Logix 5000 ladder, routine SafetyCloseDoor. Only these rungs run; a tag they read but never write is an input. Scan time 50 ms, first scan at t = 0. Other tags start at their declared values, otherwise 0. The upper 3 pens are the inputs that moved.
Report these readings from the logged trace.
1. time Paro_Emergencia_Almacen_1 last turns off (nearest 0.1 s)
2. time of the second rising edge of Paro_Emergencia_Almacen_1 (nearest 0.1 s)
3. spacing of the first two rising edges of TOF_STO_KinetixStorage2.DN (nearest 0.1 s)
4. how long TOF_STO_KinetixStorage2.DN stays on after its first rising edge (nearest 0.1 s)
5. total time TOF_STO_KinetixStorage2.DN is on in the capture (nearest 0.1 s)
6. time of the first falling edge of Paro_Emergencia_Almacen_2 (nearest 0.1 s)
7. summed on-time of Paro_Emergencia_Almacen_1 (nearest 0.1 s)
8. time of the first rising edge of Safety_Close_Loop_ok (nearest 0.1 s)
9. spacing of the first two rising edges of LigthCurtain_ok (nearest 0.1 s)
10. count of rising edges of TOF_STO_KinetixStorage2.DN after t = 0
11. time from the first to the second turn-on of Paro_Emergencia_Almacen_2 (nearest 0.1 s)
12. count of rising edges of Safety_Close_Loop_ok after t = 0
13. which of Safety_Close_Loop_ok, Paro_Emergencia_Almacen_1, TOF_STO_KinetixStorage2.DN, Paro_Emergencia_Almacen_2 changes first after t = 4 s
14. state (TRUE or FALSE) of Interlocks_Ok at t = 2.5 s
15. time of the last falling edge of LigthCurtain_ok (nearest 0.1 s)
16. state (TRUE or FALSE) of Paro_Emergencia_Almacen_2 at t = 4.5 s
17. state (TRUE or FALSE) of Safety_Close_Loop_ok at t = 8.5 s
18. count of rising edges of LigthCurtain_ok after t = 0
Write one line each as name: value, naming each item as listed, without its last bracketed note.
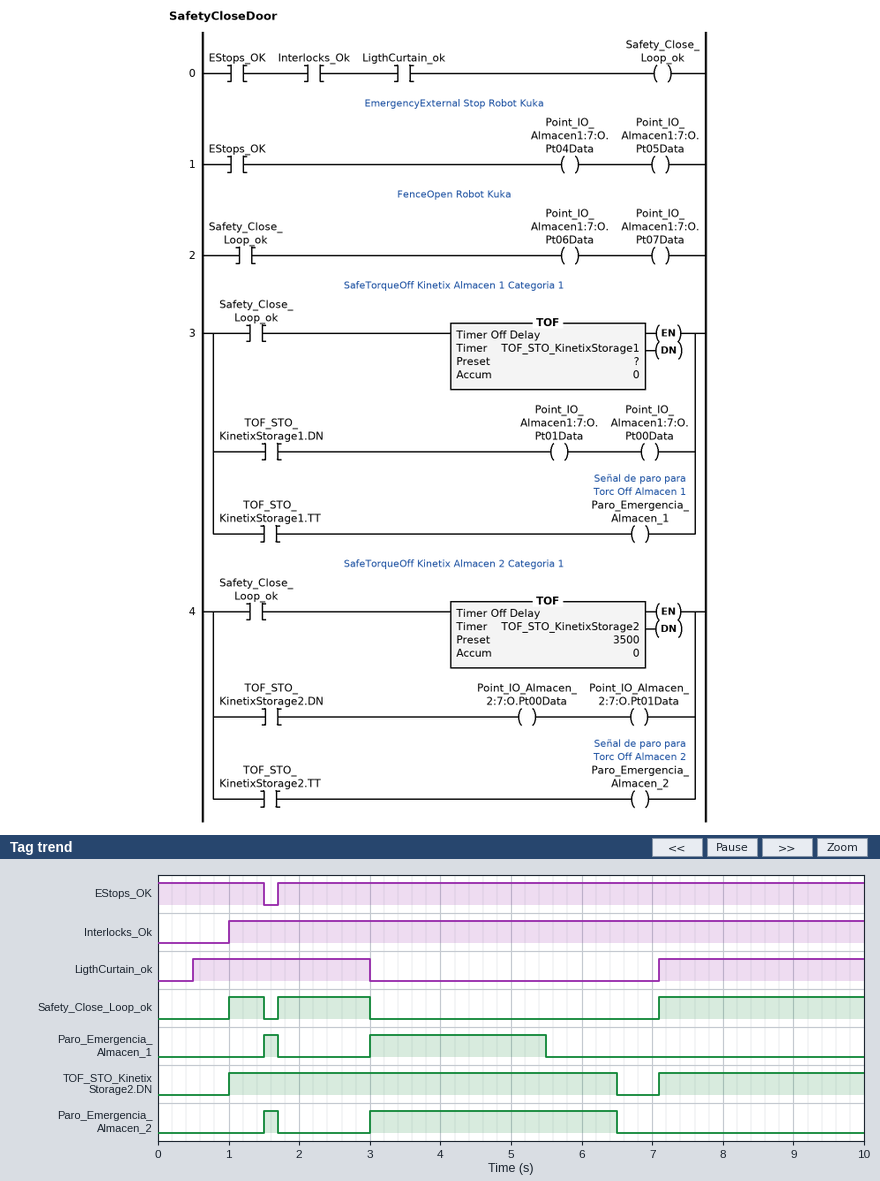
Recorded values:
time Paro_Emergencia_Almacen_1 last turns off: 5.5 s
time of the second rising edge of Paro_Emergencia_Almacen_1: 3.0 s
spacing of the first two rising edges of TOF_STO_KinetixStorage2.DN: 6.1 s
how long TOF_STO_KinetixStorage2.DN stays on after its first rising edge: 5.5 s
total time TOF_STO_KinetixStorage2.DN is on in the capture: 8.4 s
time of the first falling edge of Paro_Emergencia_Almacen_2: 1.7 s
summed on-time of Paro_Emergencia_Almacen_1: 2.7 s
time of the first rising edge of Safety_Close_Loop_ok: 1.0 s
spacing of the first two rising edges of LigthCurtain_ok: 6.6 s
count of rising edges of TOF_STO_KinetixStorage2.DN after t = 0: 2
time from the first to the second turn-on of Paro_Emergencia_Almacen_2: 1.5 s
count of rising edges of Safety_Close_Loop_ok after t = 0: 3
which of Safety_Close_Loop_ok, Paro_Emergencia_Almacen_1, TOF_STO_KinetixStorage2.DN, Paro_Emergencia_Almacen_2 changes first after t = 4 s: Paro_Emergencia_Almacen_1
state (TRUE or FALSE) of Interlocks_Ok at t = 2.5 s: TRUE
time of the last falling edge of LigthCurtain_ok: 3.0 s
state (TRUE or FALSE) of Paro_Emergencia_Almacen_2 at t = 4.5 s: TRUE
state (TRUE or FALSE) of Safety_Close_Loop_ok at t = 8.5 s: TRUE
count of rising edges of LigthCurtain_ok after t = 0: 2
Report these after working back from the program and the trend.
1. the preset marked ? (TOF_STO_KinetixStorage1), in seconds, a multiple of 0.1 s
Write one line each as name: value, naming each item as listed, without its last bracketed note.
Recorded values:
the preset marked ? (TOF_STO_KinetixStorage1), in seconds, a multiple of 0.1 s: 2.5 s
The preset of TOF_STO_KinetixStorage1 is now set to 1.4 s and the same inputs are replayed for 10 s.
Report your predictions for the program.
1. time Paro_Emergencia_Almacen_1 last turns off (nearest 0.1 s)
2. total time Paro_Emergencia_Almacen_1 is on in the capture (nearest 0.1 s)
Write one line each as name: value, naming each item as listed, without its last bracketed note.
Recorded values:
time Paro_Emergencia_Almacen_1 last turns off: 4.4 s
total time Paro_Emergencia_Almacen_1 is on in the capture: 1.6 s
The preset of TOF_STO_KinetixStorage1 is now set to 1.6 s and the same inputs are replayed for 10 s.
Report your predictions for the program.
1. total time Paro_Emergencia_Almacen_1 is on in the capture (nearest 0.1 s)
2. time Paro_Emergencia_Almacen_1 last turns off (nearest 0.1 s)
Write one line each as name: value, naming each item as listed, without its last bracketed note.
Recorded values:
total time Paro_Emergencia_Almacen_1 is on in the capture: 1.8 s
time Paro_Emergencia_Almacen_1 last turns off: 4.6 s
